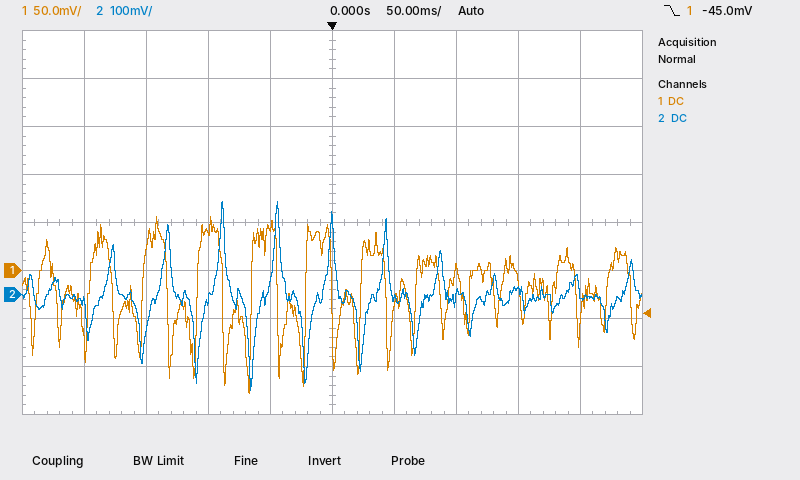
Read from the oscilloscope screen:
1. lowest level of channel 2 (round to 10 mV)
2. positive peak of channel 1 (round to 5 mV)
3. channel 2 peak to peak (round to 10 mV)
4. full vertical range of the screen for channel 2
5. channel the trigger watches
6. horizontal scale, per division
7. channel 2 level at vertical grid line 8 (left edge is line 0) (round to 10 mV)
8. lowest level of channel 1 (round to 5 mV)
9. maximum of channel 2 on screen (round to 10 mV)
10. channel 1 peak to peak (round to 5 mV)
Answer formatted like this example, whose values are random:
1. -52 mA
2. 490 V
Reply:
1. -200 mV
2. 55 mV
3. 390 mV
4. 800 mV
5. channel 1
6. 50 ms
7. 10 mV
8. -130 mV
9. 190 mV
10. 185 mV
